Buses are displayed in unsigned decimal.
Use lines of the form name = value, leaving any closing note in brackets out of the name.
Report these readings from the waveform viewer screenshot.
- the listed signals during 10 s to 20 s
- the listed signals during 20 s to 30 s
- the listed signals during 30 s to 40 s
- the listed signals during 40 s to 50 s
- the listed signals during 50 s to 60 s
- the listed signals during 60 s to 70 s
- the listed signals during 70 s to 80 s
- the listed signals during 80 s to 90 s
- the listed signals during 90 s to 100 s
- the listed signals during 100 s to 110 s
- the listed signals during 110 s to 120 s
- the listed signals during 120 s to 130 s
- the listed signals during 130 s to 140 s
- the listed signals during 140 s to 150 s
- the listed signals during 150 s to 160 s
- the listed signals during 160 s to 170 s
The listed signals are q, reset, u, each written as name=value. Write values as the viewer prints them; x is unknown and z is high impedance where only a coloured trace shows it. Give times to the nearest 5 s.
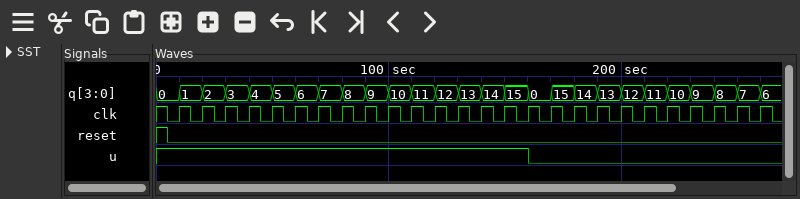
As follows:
the listed signals during 10 s to 20 s = q=1, reset=0, u=1
the listed signals during 20 s to 30 s = q=2, reset=0, u=1
the listed signals during 30 s to 40 s = q=3, reset=0, u=1
the listed signals during 40 s to 50 s = q=4, reset=0, u=1
the listed signals during 50 s to 60 s = q=5, reset=0, u=1
the listed signals during 60 s to 70 s = q=6, reset=0, u=1
the listed signals during 70 s to 80 s = q=7, reset=0, u=1
the listed signals during 80 s to 90 s = q=8, reset=0, u=1
the listed signals during 90 s to 100 s = q=9, reset=0, u=1
the listed signals during 100 s to 110 s = q=10, reset=0, u=1
the listed signals during 110 s to 120 s = q=11, reset=0, u=1
the listed signals during 120 s to 130 s = q=12, reset=0, u=1
the listed signals during 130 s to 140 s = q=13, reset=0, u=1
the listed signals during 140 s to 150 s = q=14, reset=0, u=1
the listed signals during 150 s to 160 s = q=15, reset=0, u=1
the listed signals during 160 s to 170 s = q=0, reset=0, u=0
